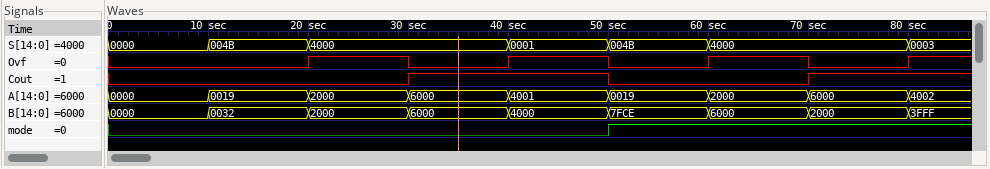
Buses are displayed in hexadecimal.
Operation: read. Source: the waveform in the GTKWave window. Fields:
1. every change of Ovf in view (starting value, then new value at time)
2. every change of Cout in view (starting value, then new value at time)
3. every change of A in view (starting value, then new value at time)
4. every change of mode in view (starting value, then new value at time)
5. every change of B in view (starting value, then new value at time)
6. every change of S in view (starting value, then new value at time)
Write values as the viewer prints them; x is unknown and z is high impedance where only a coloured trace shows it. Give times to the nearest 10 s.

0, 1 at 20 s, 0 at 30 s, 1 at 40 s, 0 at 50 s, 1 at 60 s, 0 at 70 s, 1 at 80 s
0, 1 at 30 s, 0 at 50 s, 1 at 70 s
0000, 0019 at 10 s, 2000 at 20 s, 6000 at 30 s, 4001 at 40 s, 0019 at 50 s, 2000 at 60 s, 6000 at 70 s, 4002 at 80 s
0, 1 at 50 s
0000, 0032 at 10 s, 2000 at 20 s, 6000 at 30 s, 4000 at 40 s, 7FCE at 50 s, 6000 at 60 s, 2000 at 70 s, 3FFF at 80 s
0000, 004B at 10 s, 4000 at 20 s, 0001 at 40 s, 004B at 50 s, 4000 at 60 s, 0003 at 80 s
